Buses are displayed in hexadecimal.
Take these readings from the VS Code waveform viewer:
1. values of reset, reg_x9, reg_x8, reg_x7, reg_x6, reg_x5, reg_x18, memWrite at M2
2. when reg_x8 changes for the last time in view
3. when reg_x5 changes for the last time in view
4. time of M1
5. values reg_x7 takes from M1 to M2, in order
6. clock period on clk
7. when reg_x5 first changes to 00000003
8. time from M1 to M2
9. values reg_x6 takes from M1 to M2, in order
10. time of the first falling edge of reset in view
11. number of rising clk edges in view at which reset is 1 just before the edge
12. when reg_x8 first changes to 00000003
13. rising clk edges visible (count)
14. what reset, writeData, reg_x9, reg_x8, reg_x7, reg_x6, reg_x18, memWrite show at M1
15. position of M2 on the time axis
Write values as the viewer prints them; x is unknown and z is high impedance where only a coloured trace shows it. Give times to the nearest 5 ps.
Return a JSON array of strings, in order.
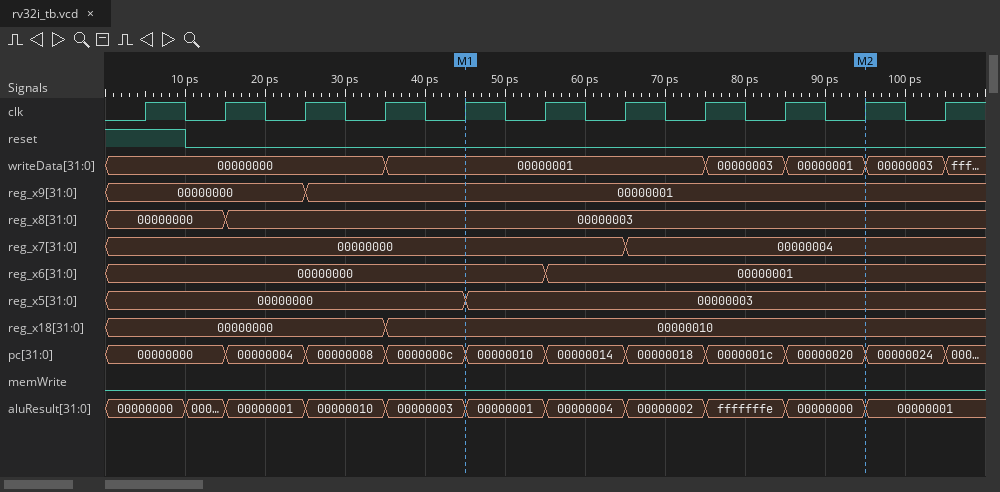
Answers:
["reset=0, reg_x9=00000001, reg_x8=00000003, reg_x7=00000004, reg_x6=00000001, reg_x5=00000003, reg_x18=00000010, memWrite=0", "15 ps", "45 ps", "45 ps", "00000000, 00000004", "10 ps", "45 ps", "50 ps", "00000000, 00000001", "10 ps", "1", "15 ps", "11", "reset=0, writeData=00000001, reg_x9=00000001, reg_x8=00000003, reg_x7=00000000, reg_x6=00000000, reg_x18=00000010, memWrite=0", "95 ps"]
